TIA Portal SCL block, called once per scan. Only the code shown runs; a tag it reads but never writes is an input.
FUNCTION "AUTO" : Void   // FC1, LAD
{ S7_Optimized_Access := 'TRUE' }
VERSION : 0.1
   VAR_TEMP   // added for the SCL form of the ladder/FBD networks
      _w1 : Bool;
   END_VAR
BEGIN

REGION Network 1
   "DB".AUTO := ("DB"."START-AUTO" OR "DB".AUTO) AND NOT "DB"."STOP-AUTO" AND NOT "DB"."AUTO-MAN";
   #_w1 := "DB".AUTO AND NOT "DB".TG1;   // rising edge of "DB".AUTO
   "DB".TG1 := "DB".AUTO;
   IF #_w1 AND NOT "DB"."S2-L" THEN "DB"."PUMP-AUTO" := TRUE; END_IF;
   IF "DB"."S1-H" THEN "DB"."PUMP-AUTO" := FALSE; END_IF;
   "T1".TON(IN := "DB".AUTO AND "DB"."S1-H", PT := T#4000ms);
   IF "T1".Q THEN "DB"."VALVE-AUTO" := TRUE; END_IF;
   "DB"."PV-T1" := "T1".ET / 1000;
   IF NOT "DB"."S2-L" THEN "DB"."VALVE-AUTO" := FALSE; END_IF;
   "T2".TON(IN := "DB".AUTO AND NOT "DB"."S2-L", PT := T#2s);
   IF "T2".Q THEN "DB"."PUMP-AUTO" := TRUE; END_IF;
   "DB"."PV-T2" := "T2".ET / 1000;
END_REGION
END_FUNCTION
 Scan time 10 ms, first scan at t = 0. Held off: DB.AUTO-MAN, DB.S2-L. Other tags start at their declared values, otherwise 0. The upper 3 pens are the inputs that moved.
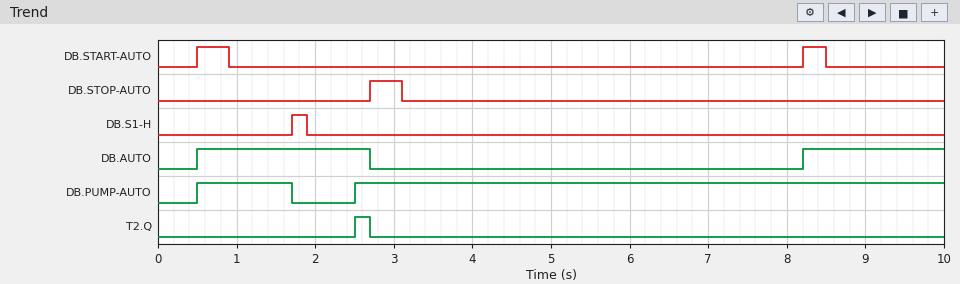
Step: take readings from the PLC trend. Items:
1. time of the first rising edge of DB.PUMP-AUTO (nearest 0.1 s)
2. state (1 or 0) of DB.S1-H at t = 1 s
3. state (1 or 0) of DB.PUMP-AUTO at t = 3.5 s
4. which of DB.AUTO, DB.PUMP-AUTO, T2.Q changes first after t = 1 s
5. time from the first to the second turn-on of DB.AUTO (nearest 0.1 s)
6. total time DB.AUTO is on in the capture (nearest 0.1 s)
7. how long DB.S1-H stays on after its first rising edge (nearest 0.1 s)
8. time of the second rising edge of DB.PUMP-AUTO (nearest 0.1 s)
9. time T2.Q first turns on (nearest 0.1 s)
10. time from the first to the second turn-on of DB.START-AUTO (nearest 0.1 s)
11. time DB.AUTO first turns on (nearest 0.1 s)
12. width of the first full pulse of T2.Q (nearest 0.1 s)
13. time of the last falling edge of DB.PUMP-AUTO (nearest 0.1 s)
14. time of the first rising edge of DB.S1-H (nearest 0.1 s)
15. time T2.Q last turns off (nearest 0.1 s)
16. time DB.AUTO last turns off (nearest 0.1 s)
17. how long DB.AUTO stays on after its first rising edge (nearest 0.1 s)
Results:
0.5 s
0
1
DB.PUMP-AUTO
7.7 s
4.0 s
0.2 s
2.5 s
2.5 s
7.7 s
0.5 s
0.2 s
1.7 s
1.7 s
2.7 s
2.7 s
2.2 s
